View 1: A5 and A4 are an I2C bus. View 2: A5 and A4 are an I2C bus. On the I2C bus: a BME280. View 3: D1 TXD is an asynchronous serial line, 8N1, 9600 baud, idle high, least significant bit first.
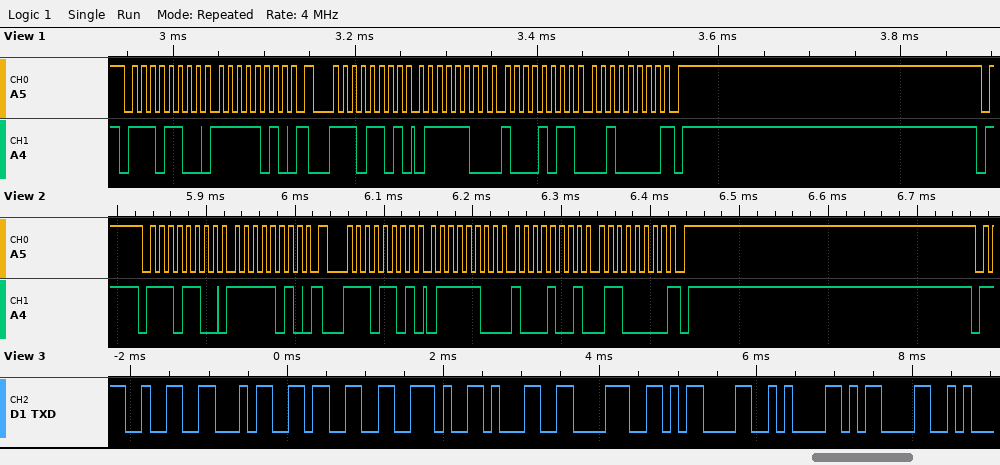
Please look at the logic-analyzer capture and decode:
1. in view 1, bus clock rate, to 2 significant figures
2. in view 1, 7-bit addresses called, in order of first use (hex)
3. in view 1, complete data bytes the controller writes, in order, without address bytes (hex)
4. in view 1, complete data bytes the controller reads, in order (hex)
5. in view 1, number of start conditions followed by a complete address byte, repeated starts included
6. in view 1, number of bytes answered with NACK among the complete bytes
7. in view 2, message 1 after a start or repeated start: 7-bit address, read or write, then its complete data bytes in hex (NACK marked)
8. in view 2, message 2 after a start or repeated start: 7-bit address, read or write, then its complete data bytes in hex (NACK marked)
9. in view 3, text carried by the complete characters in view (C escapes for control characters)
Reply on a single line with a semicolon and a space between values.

100 kHz; 0x76; FA; 7C 8B 20; 2; 1; 0x76 write: FA; 0x76 read: 7C 89 60 NACK; "243.18\r\n\r"
